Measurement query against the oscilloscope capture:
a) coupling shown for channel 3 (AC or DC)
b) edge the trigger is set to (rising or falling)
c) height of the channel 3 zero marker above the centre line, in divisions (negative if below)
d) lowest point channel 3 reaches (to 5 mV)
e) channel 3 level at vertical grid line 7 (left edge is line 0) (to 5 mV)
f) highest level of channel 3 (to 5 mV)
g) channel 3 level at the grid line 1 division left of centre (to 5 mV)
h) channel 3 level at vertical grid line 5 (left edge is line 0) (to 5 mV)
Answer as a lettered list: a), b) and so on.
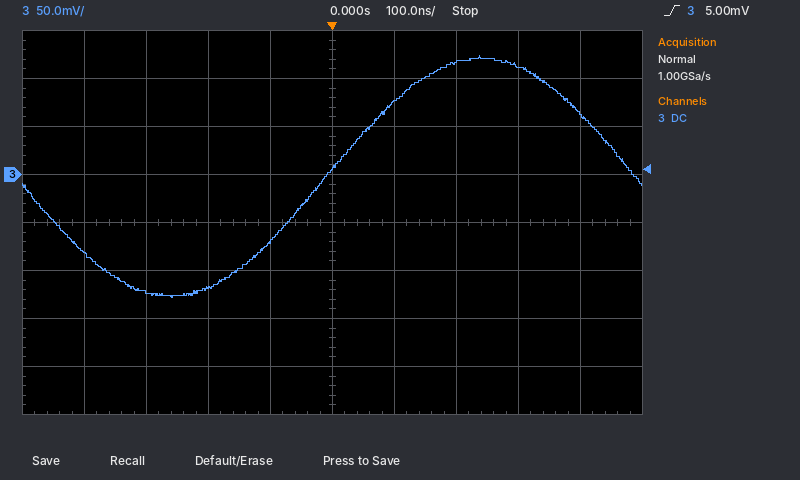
a) DC
b) rising
c) +1.0 div
d) -130 mV
e) 115 mV
f) 125 mV
g) -70 mV
h) 5 mV
